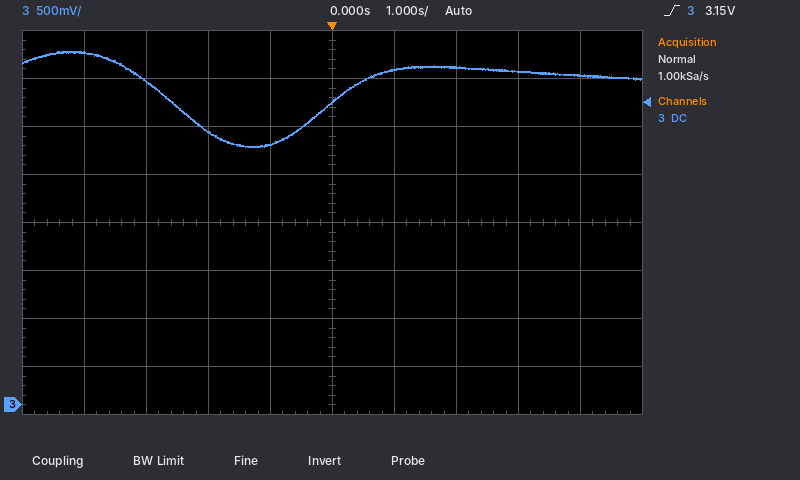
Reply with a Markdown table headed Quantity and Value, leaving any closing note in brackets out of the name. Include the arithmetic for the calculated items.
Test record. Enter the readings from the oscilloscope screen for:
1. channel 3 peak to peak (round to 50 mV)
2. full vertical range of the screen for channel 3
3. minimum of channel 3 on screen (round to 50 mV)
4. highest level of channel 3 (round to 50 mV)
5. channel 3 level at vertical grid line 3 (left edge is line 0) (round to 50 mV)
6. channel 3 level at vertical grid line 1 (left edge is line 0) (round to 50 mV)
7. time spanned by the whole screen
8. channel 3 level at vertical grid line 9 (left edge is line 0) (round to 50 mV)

| Quantity | Value |
|---|---|
| channel 3 peak to peak | 3.70 V − (2.70 V) = 1.00 V |
| full vertical range of the screen for channel 3 | 4 V |
| minimum of channel 3 on screen | 2.70 V |
| highest level of channel 3 | 3.70 V |
| channel 3 level at vertical grid line 3 (left edge is line 0) | 2.85 V |
| channel 3 level at vertical grid line 1 (left edge is line 0) | 3.65 V |
| time spanned by the whole screen | 10 s |
| channel 3 level at vertical grid line 9 (left edge is line 0) | 3.45 V |
